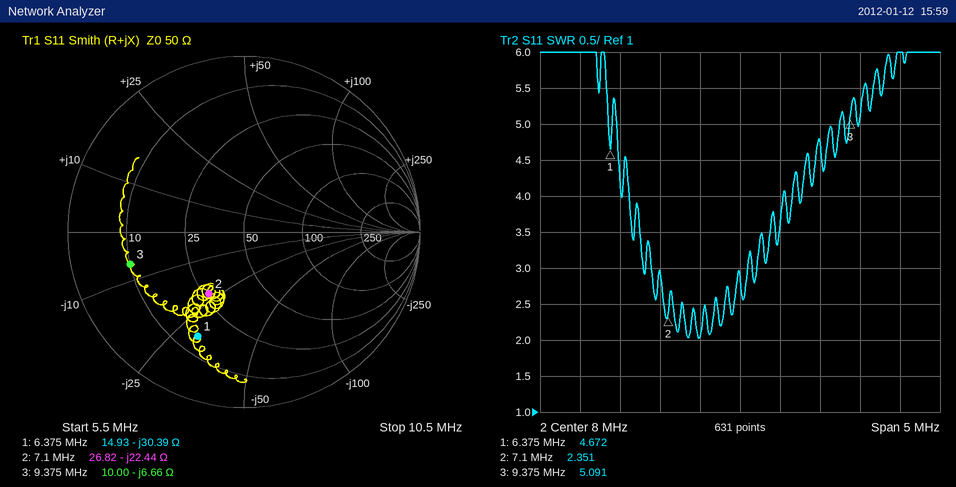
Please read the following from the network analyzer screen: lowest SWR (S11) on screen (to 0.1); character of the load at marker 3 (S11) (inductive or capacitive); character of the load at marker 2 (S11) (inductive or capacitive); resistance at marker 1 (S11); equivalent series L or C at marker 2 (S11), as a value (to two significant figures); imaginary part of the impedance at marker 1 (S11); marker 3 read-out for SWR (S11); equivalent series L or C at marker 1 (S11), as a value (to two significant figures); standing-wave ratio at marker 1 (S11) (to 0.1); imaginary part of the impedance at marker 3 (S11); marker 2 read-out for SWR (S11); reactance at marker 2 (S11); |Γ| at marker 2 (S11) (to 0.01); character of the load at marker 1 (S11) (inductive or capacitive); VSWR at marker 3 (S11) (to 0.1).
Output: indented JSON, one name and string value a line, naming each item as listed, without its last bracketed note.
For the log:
{
  "lowest SWR (S11) on screen": "2.0",
  "character of the load at marker 3 (S11)": "capacitive",
  "character of the load at marker 2 (S11)": "capacitive",
  "resistance at marker 1": "14.93 Ω",
  "equivalent series L or C at marker 2 (S11), as a value": "1.00 nF",
  "imaginary part of the impedance at marker 1": "-30.39 Ω",
  "marker 3 read-out for SWR": "5.091",
  "equivalent series L or C at marker 1 (S11), as a value": "820 pF",
  "standing-wave ratio at marker 1 (S11)": "4.7",
  "imaginary part of the impedance at marker 3": "-6.66 Ω",
  "marker 2 read-out for SWR": "2.351",
  "reactance at marker 2": "-22.44 Ω",
  "|Γ| at marker 2 (S11)": "0.40",
  "character of the load at marker 1 (S11)": "capacitive",
  "VSWR at marker 3 (S11)": "5.1"
}
